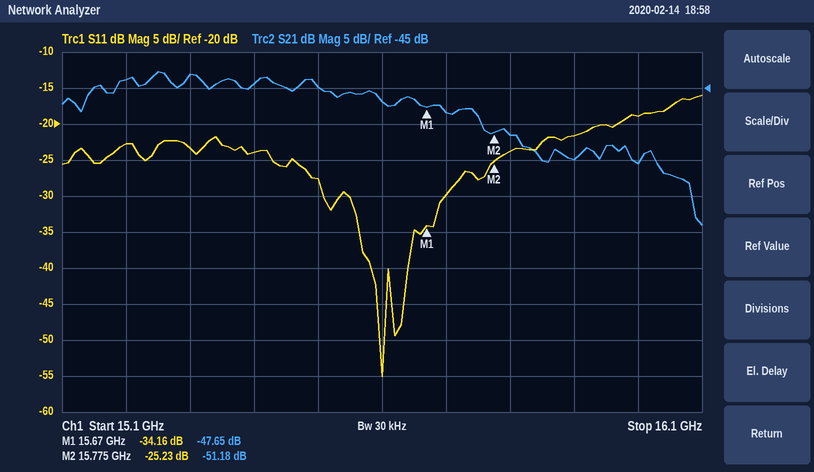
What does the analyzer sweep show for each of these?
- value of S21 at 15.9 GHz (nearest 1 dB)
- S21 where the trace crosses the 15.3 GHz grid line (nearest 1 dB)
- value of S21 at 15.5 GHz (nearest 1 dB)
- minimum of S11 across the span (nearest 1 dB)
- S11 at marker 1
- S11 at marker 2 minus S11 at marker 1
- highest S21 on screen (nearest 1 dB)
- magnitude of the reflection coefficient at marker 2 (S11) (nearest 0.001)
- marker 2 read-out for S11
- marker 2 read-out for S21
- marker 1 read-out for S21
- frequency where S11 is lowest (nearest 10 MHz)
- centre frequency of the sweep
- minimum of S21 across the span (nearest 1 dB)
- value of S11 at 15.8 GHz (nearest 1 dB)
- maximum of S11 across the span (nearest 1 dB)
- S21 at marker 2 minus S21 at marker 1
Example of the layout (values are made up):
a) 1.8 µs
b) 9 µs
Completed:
a) -55 dB
b) -43 dB
c) -45 dB
d) -55 dB
e) -34.16 dB
f) 8.93 dB
g) -43 dB
h) 0.055
i) -25.23 dB
j) -51.18 dB
k) -47.65 dB
l) 15.60 GHz
m) 15.6 GHz
n) -64 dB
o) -24 dB
p) -16 dB
q) -3.53 dB
